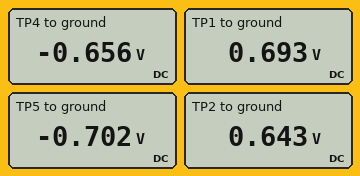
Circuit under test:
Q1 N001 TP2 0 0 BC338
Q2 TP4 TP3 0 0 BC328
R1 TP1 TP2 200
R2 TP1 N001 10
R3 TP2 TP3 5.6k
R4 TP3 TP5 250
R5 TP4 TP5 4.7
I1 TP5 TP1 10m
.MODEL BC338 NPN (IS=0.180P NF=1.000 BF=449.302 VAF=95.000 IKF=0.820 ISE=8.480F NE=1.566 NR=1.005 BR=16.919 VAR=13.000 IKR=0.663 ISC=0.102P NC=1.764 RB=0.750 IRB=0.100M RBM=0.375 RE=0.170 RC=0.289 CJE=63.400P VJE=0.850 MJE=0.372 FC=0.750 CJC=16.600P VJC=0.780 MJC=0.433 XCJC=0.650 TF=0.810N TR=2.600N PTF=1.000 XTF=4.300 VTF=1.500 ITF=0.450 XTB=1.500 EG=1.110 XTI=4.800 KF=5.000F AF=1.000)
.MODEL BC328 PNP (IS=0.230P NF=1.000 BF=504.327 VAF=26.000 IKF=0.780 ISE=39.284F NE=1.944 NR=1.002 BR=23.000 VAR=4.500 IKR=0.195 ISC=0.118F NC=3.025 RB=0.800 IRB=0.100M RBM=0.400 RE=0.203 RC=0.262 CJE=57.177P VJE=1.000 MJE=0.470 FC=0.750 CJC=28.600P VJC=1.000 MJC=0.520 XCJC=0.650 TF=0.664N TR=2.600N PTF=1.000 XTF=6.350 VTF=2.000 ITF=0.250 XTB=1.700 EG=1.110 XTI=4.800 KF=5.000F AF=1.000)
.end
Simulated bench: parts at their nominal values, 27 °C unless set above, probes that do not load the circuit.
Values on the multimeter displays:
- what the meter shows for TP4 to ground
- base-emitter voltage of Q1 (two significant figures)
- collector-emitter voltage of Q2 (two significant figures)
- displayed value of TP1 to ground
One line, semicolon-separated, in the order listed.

-0.656 V; 640 mV; -660 mV; 0.693 V
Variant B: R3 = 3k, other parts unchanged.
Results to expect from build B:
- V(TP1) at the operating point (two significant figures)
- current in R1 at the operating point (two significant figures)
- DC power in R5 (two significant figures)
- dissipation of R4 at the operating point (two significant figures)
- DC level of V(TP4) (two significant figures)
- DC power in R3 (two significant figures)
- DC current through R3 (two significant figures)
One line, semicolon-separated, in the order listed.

730 mV; 450 µA; 430 µW; 50 µW; -710 mV; 550 µW; 430 µA
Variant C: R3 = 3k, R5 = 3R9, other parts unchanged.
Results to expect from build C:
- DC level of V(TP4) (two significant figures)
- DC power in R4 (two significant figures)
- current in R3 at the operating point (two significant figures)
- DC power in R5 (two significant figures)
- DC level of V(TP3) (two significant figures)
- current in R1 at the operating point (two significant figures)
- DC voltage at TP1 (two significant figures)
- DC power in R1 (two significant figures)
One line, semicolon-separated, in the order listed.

-710 mV; 50 µW; 430 µA; 360 µW; -640 mV; 450 µA; 730 mV; 40 µW
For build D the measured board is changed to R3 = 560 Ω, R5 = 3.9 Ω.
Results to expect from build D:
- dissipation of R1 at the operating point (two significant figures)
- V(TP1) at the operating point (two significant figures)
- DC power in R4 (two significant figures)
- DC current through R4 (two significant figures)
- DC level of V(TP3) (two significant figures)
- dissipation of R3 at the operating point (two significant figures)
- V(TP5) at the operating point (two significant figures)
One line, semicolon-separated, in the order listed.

1.0 mW; 1.1 V; 1.3 mW; 2.3 mA; -630 mV; 2.9 mW; -1.2 V
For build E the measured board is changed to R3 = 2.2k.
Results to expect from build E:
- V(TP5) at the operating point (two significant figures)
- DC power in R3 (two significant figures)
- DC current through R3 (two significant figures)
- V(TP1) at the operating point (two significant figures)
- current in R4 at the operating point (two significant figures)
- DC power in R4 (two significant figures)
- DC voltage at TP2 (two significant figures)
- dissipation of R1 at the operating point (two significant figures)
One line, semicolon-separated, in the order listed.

-790 mV; 740 µW; 580 µA; 760 mV; 600 µA; 91 µW; 640 mV; 73 µW
